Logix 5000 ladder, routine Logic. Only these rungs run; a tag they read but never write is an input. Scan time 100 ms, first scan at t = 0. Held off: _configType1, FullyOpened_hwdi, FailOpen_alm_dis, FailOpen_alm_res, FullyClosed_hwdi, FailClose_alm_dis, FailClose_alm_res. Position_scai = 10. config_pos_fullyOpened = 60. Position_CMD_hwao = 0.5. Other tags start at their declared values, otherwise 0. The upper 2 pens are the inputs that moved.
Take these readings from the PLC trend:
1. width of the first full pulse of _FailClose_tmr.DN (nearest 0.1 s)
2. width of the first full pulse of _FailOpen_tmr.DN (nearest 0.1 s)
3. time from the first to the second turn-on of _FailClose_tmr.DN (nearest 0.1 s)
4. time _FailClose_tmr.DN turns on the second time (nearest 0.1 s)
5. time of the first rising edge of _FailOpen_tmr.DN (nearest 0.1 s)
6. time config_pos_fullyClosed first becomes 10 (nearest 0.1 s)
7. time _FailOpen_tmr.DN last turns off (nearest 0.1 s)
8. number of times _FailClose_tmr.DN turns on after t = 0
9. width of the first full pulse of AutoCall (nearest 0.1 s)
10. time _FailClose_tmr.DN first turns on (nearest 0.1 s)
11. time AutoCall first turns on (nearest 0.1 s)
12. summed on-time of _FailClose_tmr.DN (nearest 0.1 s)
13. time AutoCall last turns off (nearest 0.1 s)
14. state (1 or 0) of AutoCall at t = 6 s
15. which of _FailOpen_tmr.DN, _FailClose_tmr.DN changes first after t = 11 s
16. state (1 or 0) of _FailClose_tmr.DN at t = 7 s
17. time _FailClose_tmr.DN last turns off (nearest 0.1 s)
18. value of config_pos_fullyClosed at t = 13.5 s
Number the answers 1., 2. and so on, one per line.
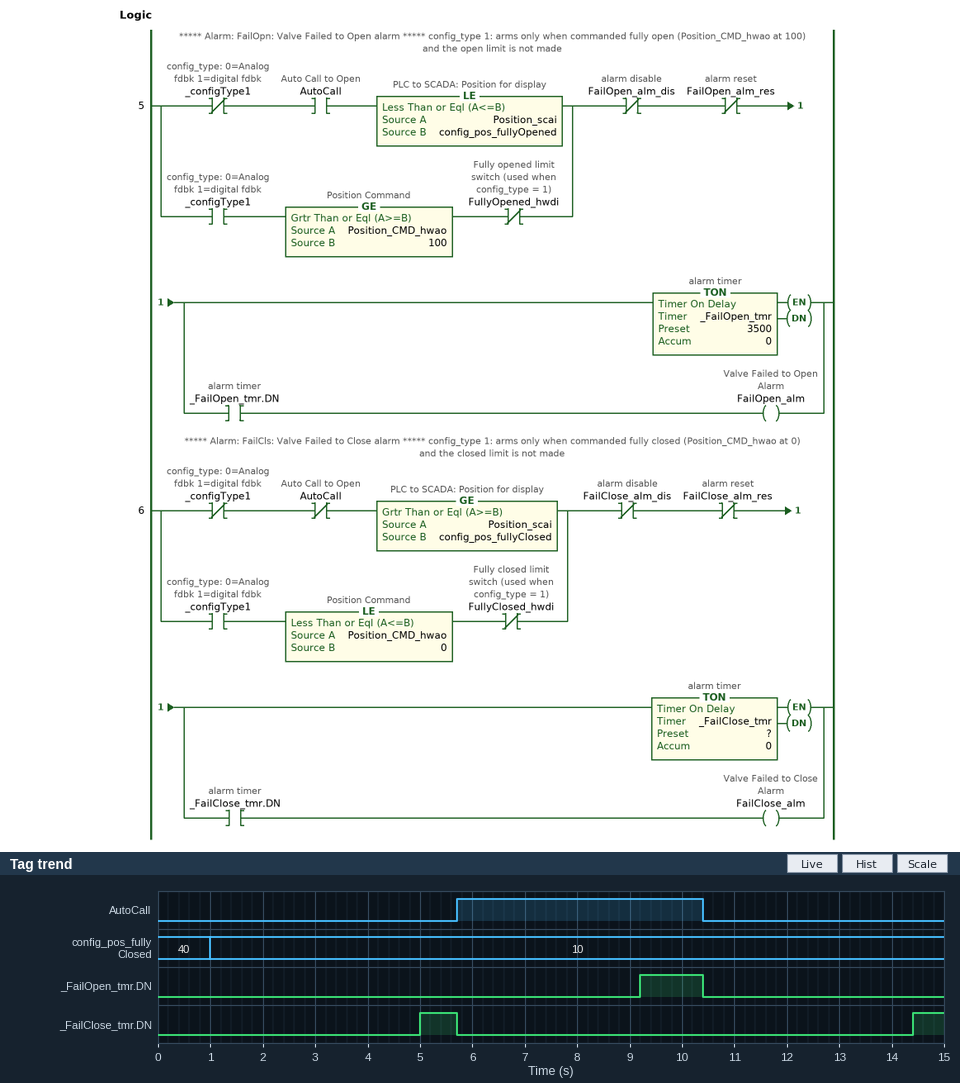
1. 0.7 s
2. 1.2 s
3. 9.4 s
4. 14.4 s
5. 9.2 s
6. 1.0 s
7. 10.4 s
8. 2
9. 4.7 s
10. 5.0 s
11. 5.7 s
12. 1.3 s
13. 10.4 s
14. 1
15. _FailClose_tmr.DN
16. 0
17. 5.7 s
18. 10
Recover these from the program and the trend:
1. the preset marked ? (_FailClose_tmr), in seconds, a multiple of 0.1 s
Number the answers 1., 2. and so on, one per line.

1. 4.0 s
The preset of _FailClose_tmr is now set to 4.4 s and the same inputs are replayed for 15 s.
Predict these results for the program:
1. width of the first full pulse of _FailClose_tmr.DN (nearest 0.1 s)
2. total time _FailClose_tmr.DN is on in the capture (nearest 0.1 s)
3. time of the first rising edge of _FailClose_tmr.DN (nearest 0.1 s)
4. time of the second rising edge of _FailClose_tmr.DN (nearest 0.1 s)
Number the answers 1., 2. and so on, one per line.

1. 0.3 s
2. 0.5 s
3. 5.4 s
4. 14.8 s
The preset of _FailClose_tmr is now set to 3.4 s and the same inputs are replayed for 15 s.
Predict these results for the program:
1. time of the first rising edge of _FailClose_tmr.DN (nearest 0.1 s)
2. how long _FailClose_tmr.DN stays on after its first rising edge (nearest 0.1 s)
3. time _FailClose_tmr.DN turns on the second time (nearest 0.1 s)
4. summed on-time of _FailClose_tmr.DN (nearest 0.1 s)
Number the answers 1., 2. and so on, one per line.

1. 4.4 s
2. 1.3 s
3. 13.8 s
4. 2.5 s
